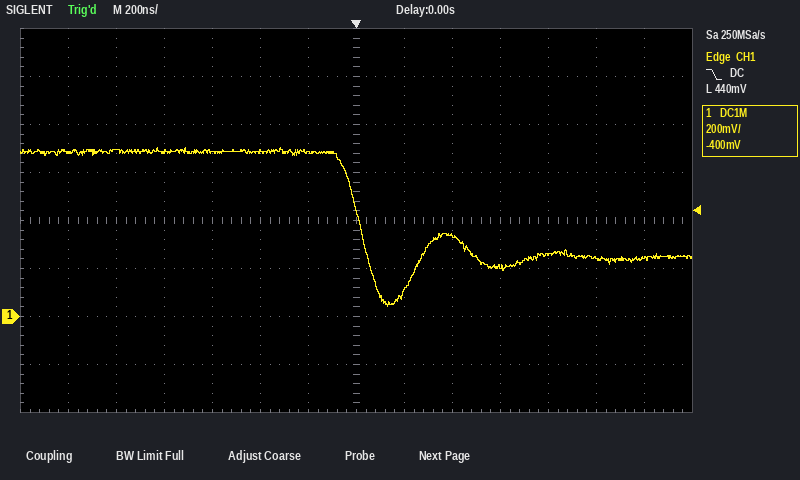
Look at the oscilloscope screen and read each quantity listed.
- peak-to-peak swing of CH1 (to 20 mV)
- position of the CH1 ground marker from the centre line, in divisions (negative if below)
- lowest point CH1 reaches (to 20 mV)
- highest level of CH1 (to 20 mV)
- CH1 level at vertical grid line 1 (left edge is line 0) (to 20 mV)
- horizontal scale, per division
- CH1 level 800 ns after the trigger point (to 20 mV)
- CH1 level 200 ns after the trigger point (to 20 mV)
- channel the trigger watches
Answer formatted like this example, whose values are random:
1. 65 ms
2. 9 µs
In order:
1. 660 mV
2. -2.0 div
3. 40 mV
4. 700 mV
5. 680 mV
6. 200 ns
7. 260 mV
8. 100 mV
9. CH1
